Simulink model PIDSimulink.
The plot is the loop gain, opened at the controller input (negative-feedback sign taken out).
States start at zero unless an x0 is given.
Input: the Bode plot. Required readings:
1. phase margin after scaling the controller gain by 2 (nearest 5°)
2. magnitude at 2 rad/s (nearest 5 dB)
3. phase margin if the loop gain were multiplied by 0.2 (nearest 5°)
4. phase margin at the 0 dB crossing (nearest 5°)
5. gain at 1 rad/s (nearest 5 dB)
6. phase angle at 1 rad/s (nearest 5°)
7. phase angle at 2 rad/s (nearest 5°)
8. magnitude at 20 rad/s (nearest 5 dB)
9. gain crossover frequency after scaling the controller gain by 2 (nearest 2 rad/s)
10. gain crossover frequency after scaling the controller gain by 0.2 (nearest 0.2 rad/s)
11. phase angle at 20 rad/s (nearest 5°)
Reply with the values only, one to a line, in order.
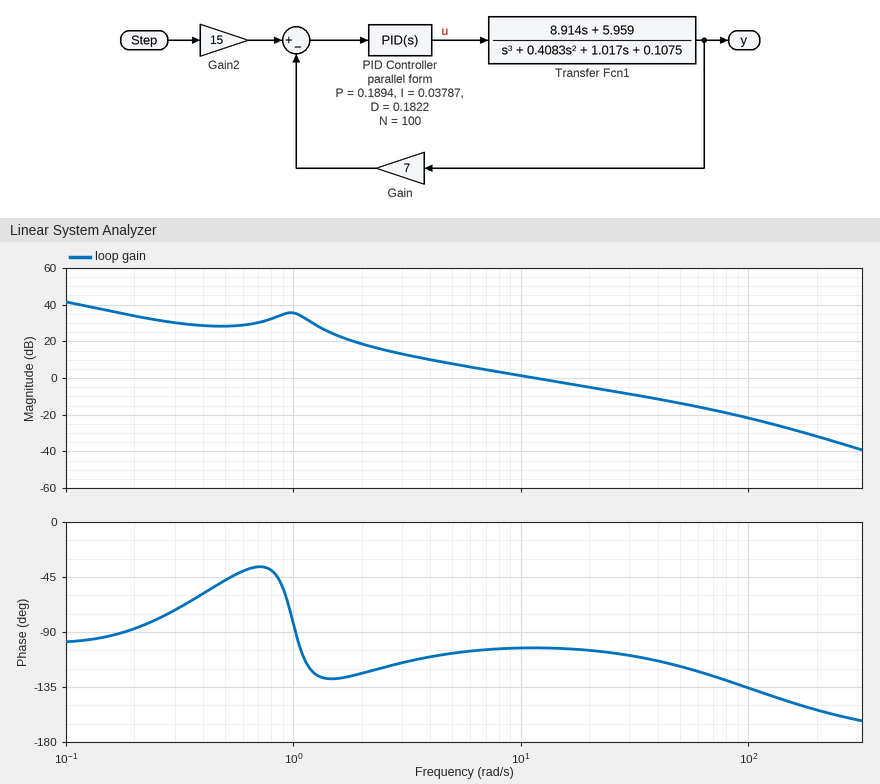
75°
20 dB
65°
75°
35 dB
-85°
-125°
-5 dB
22 rad/s
2.8 rad/s
-105°
